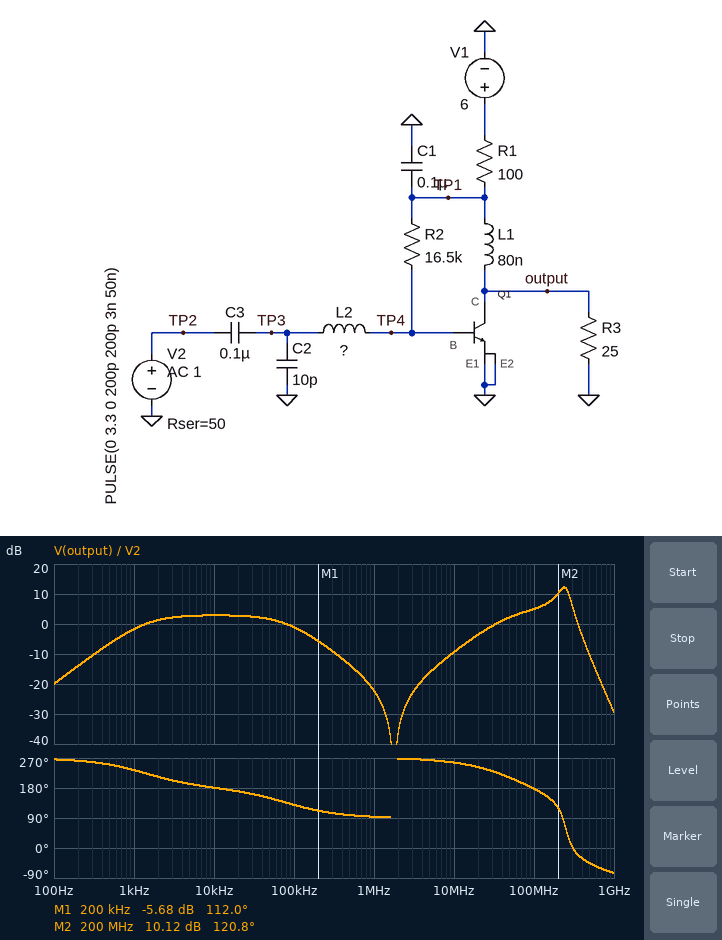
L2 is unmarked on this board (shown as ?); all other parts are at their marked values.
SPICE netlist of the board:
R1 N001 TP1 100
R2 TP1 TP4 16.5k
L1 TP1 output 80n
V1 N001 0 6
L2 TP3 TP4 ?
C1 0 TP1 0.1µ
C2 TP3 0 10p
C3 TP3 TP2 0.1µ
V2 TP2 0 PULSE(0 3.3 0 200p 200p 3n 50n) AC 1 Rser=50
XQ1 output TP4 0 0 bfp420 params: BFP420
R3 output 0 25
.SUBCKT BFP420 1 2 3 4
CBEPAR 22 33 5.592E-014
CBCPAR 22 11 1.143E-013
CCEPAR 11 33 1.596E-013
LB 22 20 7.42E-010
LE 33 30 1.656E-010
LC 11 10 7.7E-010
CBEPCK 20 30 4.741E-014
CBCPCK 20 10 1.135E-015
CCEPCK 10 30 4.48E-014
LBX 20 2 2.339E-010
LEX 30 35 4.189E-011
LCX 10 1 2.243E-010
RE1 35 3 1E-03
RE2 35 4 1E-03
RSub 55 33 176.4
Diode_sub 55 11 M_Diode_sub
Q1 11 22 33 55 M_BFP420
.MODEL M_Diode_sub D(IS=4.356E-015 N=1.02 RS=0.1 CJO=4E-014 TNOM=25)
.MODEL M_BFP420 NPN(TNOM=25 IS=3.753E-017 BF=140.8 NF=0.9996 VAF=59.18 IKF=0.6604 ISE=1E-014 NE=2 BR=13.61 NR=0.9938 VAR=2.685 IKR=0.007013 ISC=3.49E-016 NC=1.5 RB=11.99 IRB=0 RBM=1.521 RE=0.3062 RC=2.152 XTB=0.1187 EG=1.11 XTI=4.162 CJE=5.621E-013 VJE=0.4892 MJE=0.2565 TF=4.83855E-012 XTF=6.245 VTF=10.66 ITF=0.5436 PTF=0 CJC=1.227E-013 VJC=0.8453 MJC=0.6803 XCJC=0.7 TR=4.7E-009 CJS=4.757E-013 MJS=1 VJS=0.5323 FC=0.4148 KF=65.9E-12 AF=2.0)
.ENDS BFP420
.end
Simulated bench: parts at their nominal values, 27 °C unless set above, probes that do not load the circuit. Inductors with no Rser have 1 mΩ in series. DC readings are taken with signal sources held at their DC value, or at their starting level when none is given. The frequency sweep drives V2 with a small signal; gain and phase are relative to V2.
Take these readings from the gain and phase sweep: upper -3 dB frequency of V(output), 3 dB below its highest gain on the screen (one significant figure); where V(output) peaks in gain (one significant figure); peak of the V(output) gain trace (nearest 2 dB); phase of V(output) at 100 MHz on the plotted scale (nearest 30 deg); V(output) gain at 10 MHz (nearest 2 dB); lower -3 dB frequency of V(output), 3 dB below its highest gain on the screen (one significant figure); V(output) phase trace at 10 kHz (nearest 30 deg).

300 MHz
200 MHz
12 dB
180 deg
-10 dB
200 MHz
180 deg
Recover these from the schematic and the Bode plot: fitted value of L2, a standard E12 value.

220 nH
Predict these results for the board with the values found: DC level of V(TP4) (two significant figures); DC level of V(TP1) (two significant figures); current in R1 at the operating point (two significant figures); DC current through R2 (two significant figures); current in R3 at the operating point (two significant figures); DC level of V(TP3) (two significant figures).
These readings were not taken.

820 mV
1.2 V
48 mA
21 µA
46 mA
820 mV
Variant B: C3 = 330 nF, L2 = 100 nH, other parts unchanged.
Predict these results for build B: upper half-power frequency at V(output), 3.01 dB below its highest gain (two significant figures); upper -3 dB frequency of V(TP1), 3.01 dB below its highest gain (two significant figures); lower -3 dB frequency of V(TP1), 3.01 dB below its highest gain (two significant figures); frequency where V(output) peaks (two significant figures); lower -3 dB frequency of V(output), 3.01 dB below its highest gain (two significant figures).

410 MHz
81 kHz
420 Hz
360 MHz
300 MHz
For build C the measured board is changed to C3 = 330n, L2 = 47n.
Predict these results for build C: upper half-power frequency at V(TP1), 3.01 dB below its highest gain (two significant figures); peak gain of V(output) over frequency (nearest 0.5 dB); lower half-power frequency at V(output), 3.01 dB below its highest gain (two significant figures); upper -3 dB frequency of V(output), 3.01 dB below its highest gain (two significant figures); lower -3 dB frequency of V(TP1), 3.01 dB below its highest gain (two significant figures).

81 kHz
11.0 dB
450 MHz
590 MHz
420 Hz
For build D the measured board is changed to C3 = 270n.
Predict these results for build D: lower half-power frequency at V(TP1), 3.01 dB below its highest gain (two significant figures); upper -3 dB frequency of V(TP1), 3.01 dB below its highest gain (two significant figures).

510 Hz
81 kHz
